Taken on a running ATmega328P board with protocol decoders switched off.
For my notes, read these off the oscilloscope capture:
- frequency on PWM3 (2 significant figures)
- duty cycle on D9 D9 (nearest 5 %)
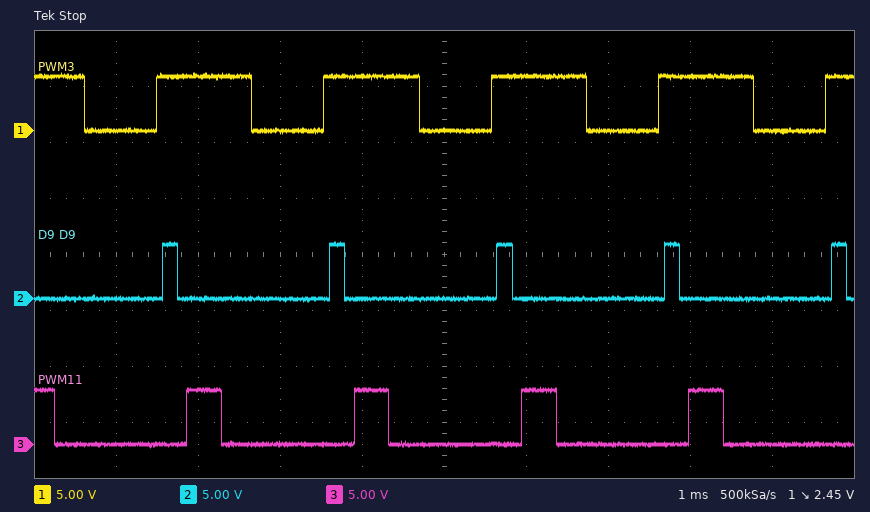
490 Hz
10 %
